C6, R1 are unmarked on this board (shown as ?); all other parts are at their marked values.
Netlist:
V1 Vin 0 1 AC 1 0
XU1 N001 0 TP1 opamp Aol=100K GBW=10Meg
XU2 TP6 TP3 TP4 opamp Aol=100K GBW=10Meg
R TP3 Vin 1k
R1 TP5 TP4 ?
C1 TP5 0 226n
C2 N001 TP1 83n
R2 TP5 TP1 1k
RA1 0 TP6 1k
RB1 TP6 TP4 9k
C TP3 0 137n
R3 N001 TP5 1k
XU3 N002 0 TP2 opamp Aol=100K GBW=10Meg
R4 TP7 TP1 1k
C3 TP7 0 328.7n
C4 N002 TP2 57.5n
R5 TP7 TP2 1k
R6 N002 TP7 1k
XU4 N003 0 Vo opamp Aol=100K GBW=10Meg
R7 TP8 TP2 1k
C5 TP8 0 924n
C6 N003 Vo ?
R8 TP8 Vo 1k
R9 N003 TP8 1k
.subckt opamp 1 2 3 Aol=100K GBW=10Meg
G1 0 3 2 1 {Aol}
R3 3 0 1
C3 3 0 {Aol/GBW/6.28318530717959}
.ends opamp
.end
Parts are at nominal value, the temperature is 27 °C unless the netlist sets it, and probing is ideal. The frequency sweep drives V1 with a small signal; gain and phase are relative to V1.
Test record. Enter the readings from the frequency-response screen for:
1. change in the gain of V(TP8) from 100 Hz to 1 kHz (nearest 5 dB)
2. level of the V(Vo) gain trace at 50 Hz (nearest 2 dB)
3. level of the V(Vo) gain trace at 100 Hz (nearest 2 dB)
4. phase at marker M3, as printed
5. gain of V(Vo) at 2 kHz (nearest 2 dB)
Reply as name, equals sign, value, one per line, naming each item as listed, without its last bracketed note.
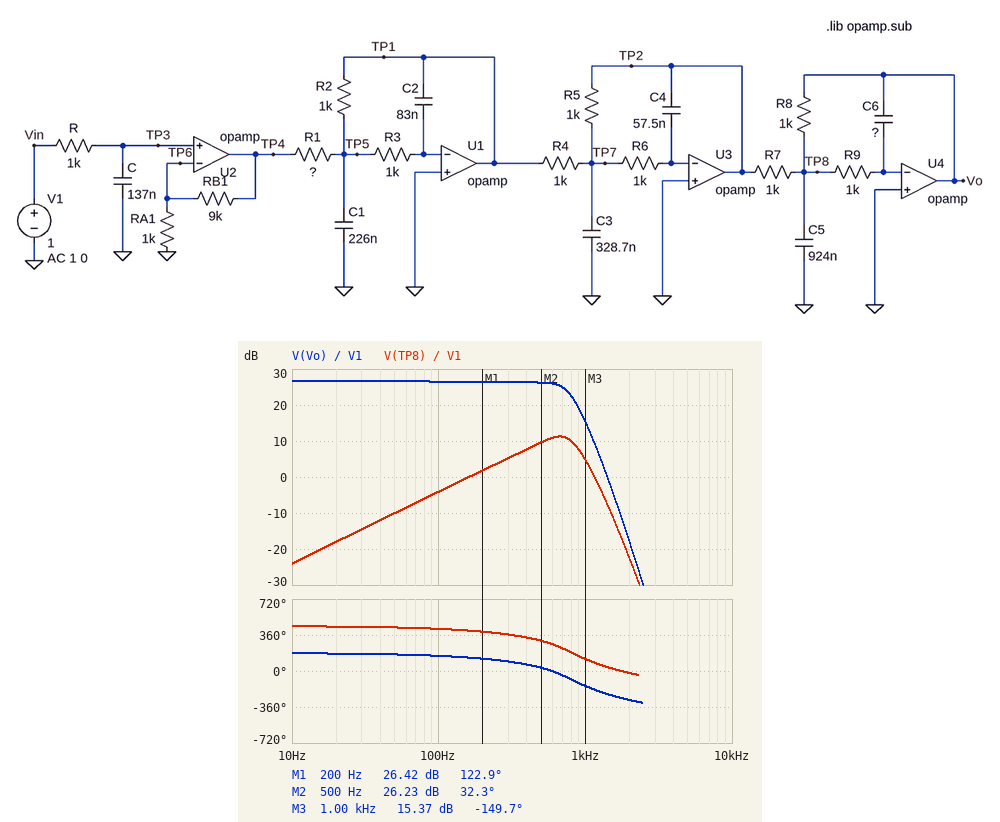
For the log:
change in the gain of V(TP8) from 100 Hz to 1 kHz = 10 dB
level of the V(Vo) gain trace at 50 Hz = 26 dB
level of the V(Vo) gain trace at 100 Hz = 26 dB
phase at marker M3, as printed = -149.7 deg
gain of V(Vo) at 2 kHz = -18 dB
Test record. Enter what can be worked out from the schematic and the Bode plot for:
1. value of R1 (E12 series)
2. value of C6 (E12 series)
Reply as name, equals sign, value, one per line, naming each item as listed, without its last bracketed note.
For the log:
value of R1 = 470 Ω
value of C6 = 47 nF
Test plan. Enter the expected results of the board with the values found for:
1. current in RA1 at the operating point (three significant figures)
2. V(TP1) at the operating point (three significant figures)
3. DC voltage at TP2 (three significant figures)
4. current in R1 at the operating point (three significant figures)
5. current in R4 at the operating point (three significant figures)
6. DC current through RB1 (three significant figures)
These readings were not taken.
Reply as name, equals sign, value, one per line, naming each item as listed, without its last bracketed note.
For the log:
current in RA1 at the operating point = 1.00 mA
V(TP1) at the operating point = -21.3 V
DC voltage at TP2 = 21.3 V
current in R1 at the operating point = 21.3 mA
current in R4 at the operating point = 21.3 mA
DC current through RB1 = 1.00 mA
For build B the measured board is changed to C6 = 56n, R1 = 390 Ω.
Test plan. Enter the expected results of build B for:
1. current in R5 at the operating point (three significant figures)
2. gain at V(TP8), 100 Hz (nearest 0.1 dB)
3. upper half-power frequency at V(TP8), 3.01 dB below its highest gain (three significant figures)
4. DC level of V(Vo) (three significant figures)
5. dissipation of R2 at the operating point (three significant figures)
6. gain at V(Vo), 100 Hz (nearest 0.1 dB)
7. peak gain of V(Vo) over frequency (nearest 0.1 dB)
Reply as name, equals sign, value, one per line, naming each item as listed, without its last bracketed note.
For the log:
current in R5 at the operating point = 25.6 mA
gain at V(TP8), 100 Hz = -1.0 dB
upper half-power frequency at V(TP8), 3.01 dB below its highest gain = 816 Hz
DC level of V(Vo) = -25.6 V
dissipation of R2 at the operating point = 657 mW
gain at V(Vo), 100 Hz = 28.1 dB
peak gain of V(Vo) over frequency = 28.2 dB
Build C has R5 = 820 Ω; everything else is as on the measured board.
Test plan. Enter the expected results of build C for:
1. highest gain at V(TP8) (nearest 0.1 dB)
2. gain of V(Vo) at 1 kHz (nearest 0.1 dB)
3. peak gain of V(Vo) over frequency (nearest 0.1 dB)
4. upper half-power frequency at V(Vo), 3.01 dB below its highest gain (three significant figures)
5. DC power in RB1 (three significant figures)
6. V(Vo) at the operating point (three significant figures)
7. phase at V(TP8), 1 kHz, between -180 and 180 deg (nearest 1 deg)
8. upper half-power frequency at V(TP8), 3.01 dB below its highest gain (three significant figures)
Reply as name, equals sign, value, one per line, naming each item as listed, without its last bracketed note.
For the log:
highest gain at V(TP8) = 9.7 dB
gain of V(Vo) at 1 kHz = 14.3 dB
peak gain of V(Vo) over frequency = 24.8 dB
upper half-power frequency at V(Vo), 3.01 dB below its highest gain = 775 Hz
DC power in RB1 = 9.00 mW
V(Vo) at the operating point = -17.4 V
phase at V(TP8), 1 kHz, between -180 and 180 deg = 129 deg
upper half-power frequency at V(TP8), 3.01 dB below its highest gain = 889 Hz
